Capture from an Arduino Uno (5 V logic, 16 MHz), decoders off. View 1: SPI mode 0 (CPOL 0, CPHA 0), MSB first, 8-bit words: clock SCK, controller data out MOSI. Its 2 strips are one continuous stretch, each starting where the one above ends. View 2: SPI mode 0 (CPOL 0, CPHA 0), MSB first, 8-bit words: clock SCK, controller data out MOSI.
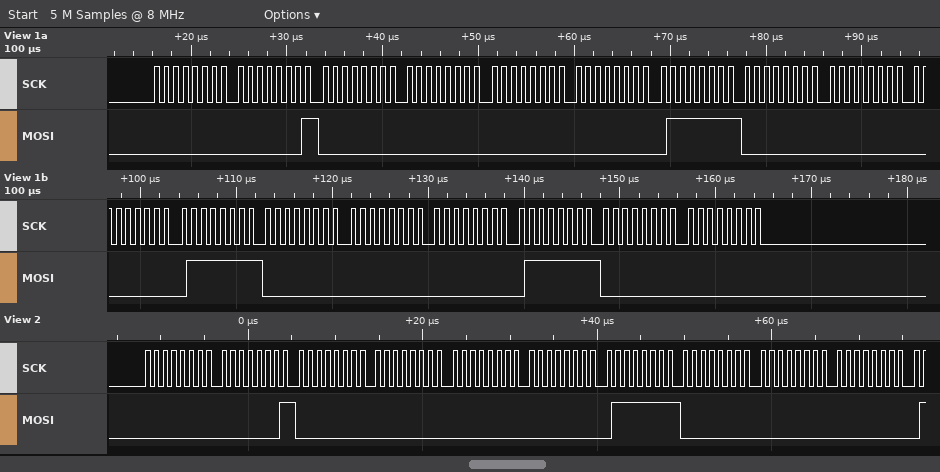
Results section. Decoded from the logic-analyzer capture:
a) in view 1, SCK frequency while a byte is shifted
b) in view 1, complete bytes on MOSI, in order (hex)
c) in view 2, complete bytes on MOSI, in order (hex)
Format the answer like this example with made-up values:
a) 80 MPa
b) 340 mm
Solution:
a) 1 MHz
b) 00 01 00 00 00 00 7F 00 00 00 7F 00 00 00 7F 00 00
c) 00 01 00 00 00 00 7F 00 00 00
